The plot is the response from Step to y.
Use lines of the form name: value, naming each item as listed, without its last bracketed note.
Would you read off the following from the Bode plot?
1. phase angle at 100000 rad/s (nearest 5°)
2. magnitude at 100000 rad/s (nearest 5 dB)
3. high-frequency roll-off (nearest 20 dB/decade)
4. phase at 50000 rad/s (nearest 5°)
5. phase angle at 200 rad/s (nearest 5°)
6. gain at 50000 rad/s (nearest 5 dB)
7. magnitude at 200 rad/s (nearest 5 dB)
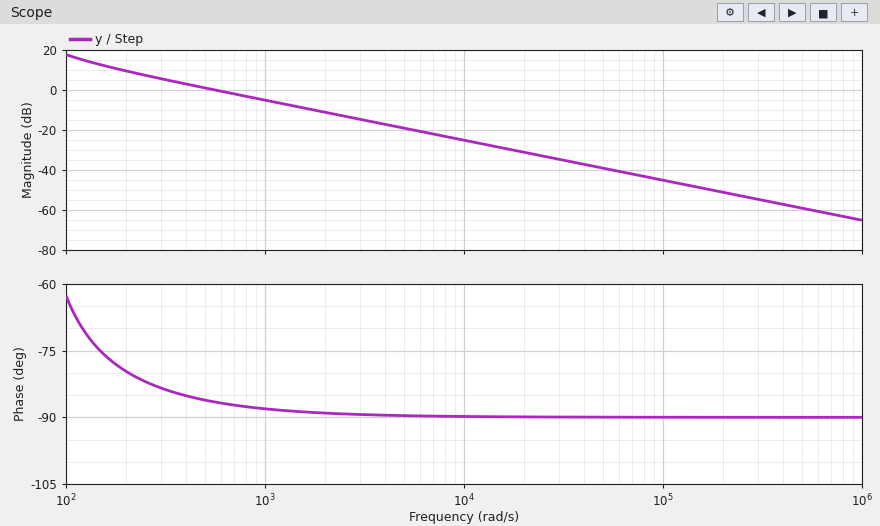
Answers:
phase angle at 100000 rad/s: -90°
magnitude at 100000 rad/s: -45 dB
high-frequency roll-off: -20 dB/decade
phase at 50000 rad/s: -90°
phase angle at 200 rad/s: -80°
gain at 50000 rad/s: -40 dB
magnitude at 200 rad/s: 10 dB
